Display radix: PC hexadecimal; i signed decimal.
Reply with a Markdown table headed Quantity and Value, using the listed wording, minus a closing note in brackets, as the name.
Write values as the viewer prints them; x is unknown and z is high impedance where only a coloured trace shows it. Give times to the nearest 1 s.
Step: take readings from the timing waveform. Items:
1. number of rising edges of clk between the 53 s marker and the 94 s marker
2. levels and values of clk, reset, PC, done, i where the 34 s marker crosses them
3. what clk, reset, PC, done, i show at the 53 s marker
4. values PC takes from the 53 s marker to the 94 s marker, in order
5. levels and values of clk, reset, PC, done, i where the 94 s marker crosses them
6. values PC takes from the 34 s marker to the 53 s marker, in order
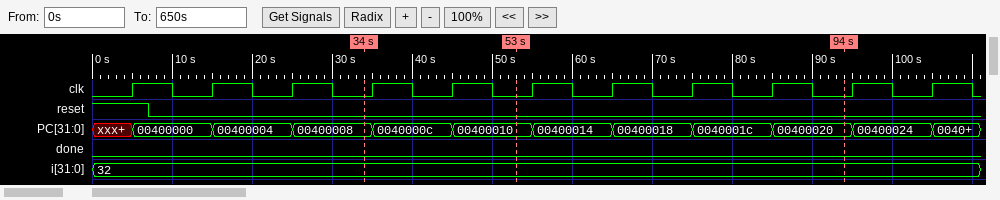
| Quantity | Value |
|---|---|
| number of rising edges of clk between the 53 s marker and the 94 s marker | 4 |
| levels and values of clk, reset, PC, done, i where the 34 s marker crosses them | clk=0, reset=0, PC=00400008, done=0, i=32 |
| what clk, reset, PC, done, i show at the 53 s marker | clk=0, reset=0, PC=00400010, done=0, i=32 |
| values PC takes from the 53 s marker to the 94 s marker, in order | 00400010, 00400014, 00400018, 0040001c, 00400020 |
| levels and values of clk, reset, PC, done, i where the 94 s marker crosses them | clk=0, reset=0, PC=00400020, done=0, i=32 |
| values PC takes from the 34 s marker to the 53 s marker, in order | 00400008, 0040000c, 00400010 |
